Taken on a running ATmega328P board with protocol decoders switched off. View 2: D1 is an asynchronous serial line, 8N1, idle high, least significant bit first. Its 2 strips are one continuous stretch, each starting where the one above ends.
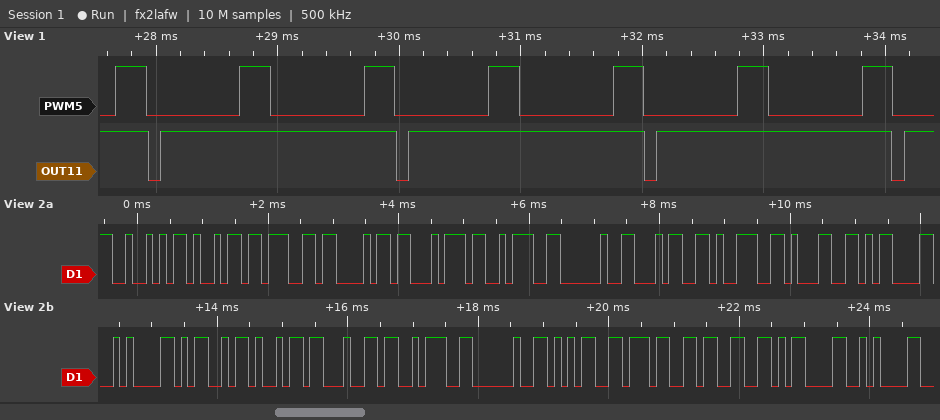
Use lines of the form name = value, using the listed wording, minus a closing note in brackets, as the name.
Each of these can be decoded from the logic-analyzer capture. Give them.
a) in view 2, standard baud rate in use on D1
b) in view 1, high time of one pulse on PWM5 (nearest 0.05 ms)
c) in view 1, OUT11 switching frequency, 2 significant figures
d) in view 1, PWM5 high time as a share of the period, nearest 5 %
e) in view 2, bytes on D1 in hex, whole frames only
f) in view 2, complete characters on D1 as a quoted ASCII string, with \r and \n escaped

in view 2, standard baud rate in use on D1 = 9600 baud
in view 1, high time of one pulse on PWM5 = 0.25 ms
in view 1, OUT11 switching frequency, 2 significant figures = 490 Hz
in view 1, PWM5 high time as a share of the period, nearest 5 % = 25 %
in view 2, bytes on D1 in hex, whole frames only = 52 69 67 68 74 3A 20 34 39 31 0D 0A 4D 69 64 3A 20 35 37 33 0D 0A
in view 2, complete characters on D1 as a quoted ASCII string, with \r and \n escaped = "Right: 491\r\nMid: 573\r\n"
